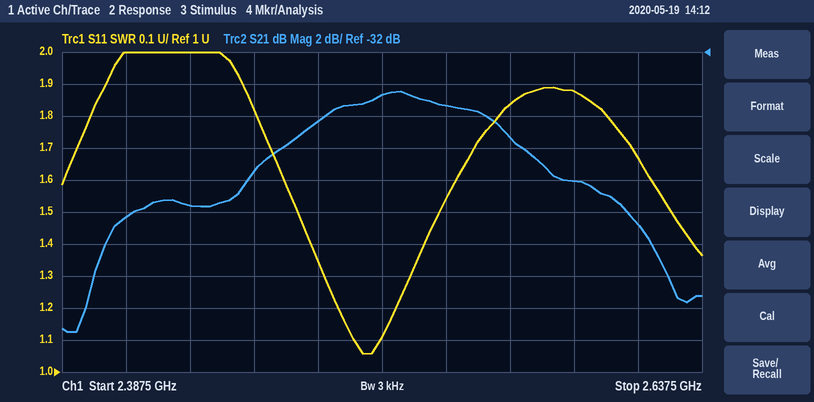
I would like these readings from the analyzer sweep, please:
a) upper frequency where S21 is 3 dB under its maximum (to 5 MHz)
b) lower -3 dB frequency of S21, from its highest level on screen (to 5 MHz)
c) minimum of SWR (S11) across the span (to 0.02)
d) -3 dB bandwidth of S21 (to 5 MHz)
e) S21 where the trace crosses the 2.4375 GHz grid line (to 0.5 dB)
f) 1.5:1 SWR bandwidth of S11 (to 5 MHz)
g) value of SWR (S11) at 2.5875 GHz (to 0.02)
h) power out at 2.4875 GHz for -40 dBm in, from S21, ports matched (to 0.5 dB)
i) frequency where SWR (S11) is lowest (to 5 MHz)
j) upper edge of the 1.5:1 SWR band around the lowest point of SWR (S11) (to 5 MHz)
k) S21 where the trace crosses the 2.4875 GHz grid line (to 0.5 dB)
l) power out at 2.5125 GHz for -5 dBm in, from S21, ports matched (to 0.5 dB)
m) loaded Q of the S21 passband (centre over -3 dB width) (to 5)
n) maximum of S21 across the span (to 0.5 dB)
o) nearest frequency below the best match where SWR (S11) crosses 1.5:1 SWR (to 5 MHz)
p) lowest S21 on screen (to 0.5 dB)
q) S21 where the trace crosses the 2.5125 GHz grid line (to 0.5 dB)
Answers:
2.565 GHz
2.480 GHz
1.06
85 MHz
-41.5 dB
55 MHz
1.88
-76.5 dBm
2.505 GHz
2.535 GHz
-36.5 dB
-39.5 dBm
30
-34.5 dB
2.480 GHz
-49.5 dB
-34.5 dB
